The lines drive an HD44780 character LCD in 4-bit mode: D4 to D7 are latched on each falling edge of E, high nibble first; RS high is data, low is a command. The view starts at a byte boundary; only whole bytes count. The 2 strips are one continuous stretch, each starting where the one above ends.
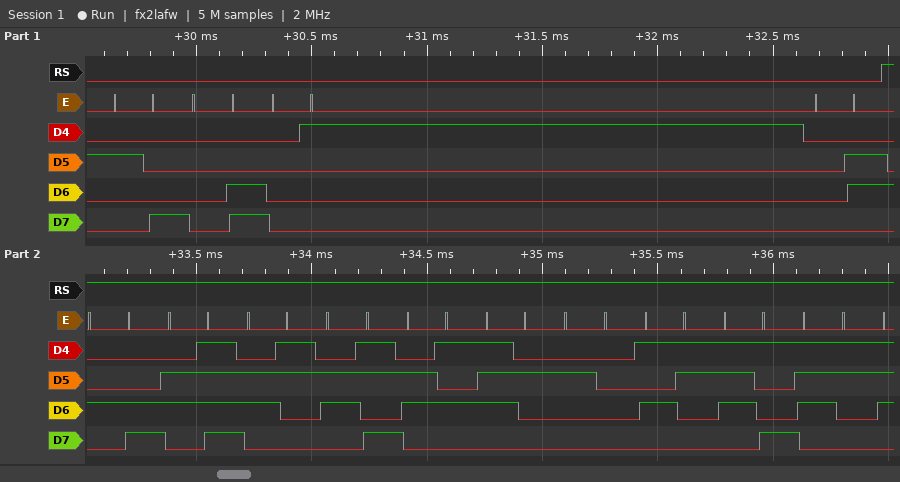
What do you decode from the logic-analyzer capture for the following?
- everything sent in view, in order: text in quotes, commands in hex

0x28 0x0C 0x01 0x06 "Locker Sys"
